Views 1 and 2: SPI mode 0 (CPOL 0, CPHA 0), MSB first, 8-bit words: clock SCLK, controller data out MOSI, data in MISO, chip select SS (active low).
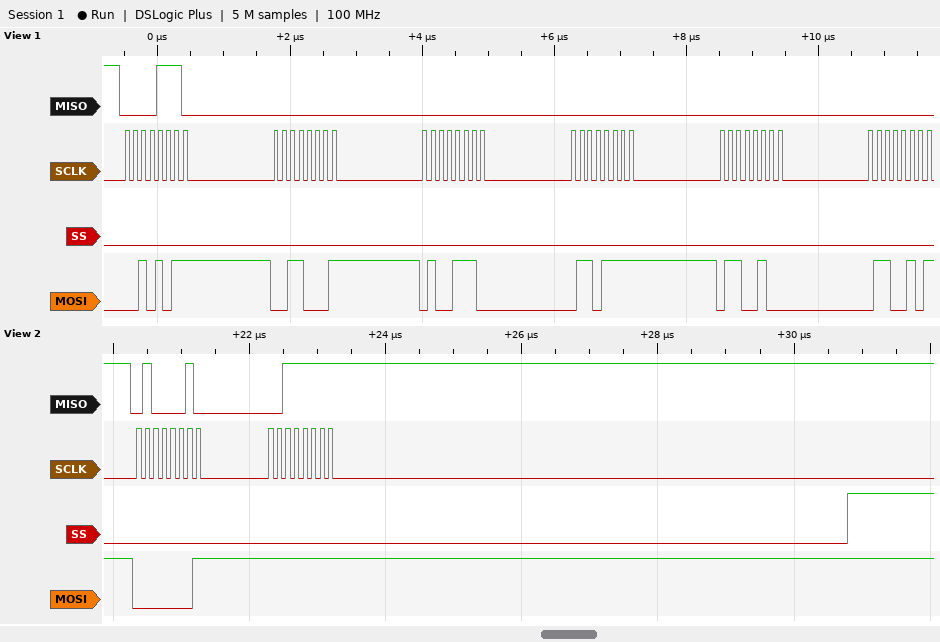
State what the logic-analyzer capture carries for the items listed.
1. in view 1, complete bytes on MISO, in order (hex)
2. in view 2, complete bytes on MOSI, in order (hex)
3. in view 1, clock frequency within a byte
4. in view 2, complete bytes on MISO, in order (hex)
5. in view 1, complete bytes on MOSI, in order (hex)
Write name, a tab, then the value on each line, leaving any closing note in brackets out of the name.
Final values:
in view 1, complete bytes on MISO, in order	0E 00 00 00 00 00
in view 2, complete bytes on MOSI, in order	0x01 0xFF
in view 1, clock frequency within a byte	8 MHz
in view 2, complete bytes on MISO, in order	0x42 0x3F
in view 1, complete bytes on MOSI, in order	2B 31 4E 6F 64 65
